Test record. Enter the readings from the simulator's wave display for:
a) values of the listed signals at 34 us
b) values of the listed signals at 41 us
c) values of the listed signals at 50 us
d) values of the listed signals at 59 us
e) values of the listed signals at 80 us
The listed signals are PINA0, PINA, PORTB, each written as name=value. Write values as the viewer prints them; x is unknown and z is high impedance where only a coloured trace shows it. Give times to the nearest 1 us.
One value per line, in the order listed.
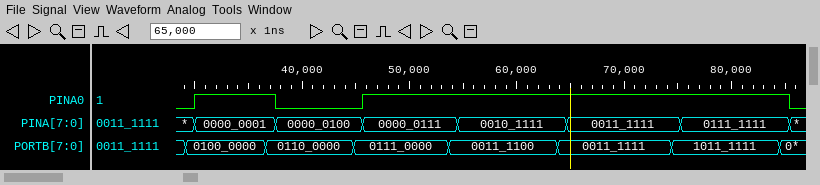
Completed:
PINA0=1, PINA=0000_0001, PORTB=0100_0000
PINA0=0, PINA=0000_0100, PORTB=0110_0000
PINA0=1, PINA=0000_0111, PORTB=0111_0000
PINA0=1, PINA=0010_1111, PORTB=0011_1100
PINA0=1, PINA=0111_1111, PORTB=1011_1111
